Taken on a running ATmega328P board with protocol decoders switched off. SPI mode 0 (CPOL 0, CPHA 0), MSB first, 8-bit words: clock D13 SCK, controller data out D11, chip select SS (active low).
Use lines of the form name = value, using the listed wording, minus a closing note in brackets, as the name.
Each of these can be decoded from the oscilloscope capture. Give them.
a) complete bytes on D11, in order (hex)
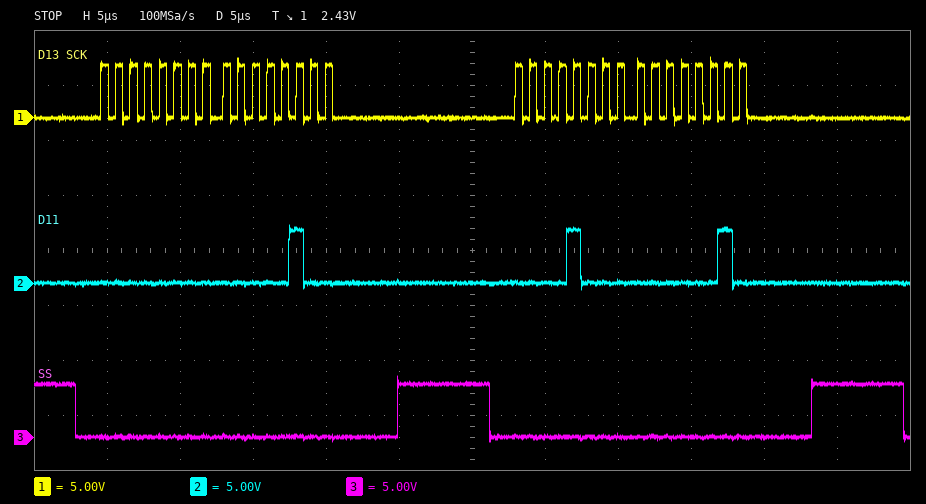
complete bytes on D11, in order = 00 04 08 02
